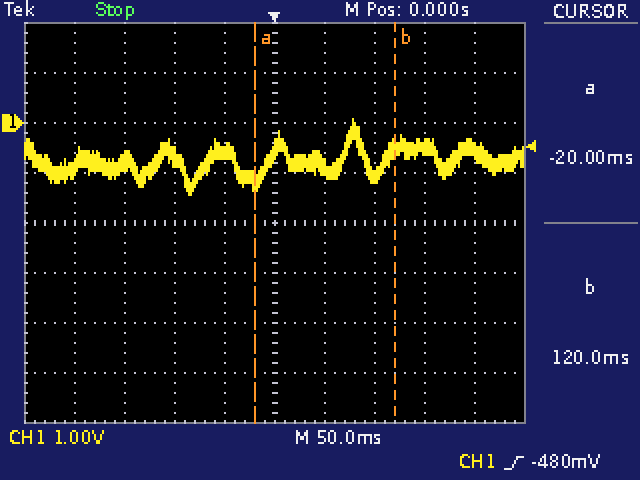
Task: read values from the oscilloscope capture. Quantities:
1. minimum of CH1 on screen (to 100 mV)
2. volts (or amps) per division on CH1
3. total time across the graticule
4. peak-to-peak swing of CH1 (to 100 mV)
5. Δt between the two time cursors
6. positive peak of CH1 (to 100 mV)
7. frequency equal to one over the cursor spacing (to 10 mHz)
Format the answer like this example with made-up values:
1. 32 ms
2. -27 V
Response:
1. -1.4 V
2. 1 V
3. 500 ms
4. 1.5 V
5. 140 ms
6. 100 mV
7. 7.14 Hz
